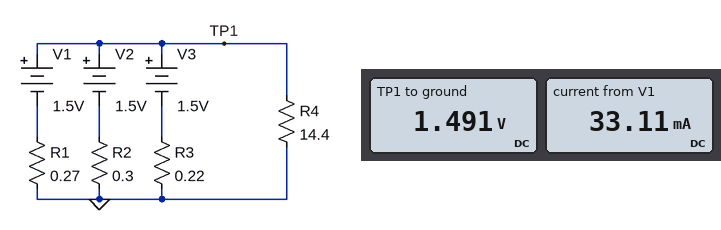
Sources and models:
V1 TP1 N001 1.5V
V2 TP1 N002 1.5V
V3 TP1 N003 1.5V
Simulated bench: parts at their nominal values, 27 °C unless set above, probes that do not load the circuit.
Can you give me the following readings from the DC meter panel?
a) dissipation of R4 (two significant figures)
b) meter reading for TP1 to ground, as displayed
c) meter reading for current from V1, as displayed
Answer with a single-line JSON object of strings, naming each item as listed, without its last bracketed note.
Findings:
{"dissipation of R4": "150 mW", "meter reading for TP1 to ground, as displayed": "1.491 V", "meter reading for current from V1, as displayed": "33.11 mA"}
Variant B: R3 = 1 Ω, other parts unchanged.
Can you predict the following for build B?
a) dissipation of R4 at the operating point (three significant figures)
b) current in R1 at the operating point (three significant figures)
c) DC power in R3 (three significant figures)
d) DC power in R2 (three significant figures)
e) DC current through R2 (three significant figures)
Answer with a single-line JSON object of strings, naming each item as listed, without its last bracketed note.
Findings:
{"dissipation of R4 at the operating point": "154 mW", "current in R1 at the operating point": "47.6 mA", "DC power in R3": "165 µW", "DC power in R2": "550 µW", "DC current through R2": "42.8 mA"}
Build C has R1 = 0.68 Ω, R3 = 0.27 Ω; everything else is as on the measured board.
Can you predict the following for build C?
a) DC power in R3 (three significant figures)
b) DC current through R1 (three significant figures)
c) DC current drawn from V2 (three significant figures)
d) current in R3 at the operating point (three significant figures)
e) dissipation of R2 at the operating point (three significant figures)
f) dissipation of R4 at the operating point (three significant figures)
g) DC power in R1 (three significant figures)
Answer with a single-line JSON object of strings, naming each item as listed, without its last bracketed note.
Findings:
{"DC power in R3": "546 µW", "DC current through R1": "17.9 mA", "DC current drawn from V2": "40.5 mA", "current in R3 at the operating point": "45.0 mA", "dissipation of R2 at the operating point": "492 µW", "dissipation of R4 at the operating point": "154 mW", "DC power in R1": "217 µW"}
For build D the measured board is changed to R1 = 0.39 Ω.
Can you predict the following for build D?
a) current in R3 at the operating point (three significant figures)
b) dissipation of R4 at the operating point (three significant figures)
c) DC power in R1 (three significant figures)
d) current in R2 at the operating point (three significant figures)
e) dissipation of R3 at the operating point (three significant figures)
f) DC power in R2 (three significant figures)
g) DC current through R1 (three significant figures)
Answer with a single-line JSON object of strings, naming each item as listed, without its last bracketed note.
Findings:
{"current in R3 at the operating point": "45.0 mA", "dissipation of R4 at the operating point": "154 mW", "DC power in R1": "252 µW", "current in R2 at the operating point": "33.0 mA", "dissipation of R3 at the operating point": "446 µW", "DC power in R2": "327 µW", "DC current through R1": "25.4 mA"}
